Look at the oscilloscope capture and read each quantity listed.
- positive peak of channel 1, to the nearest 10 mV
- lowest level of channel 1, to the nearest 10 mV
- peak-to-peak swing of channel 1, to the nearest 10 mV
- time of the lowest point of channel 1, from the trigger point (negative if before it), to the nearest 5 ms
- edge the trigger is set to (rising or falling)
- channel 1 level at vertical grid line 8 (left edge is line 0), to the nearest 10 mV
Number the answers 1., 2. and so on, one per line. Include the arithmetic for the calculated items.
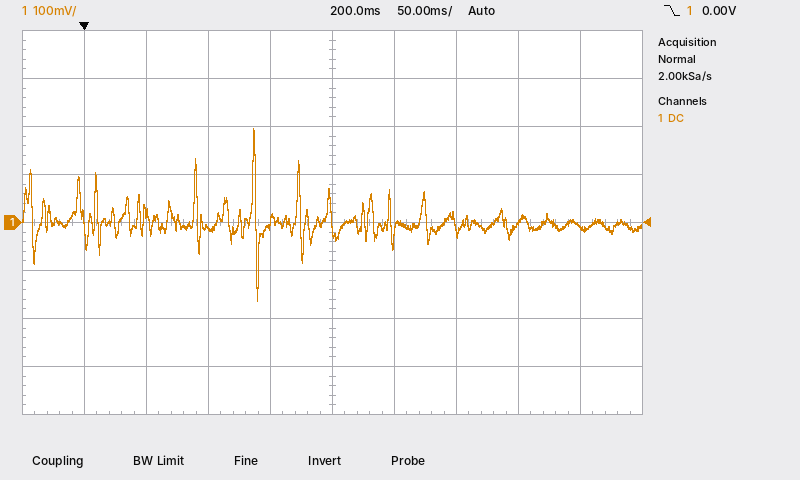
1. 200 mV
2. -160 mV
3. 200 mV − (-160 mV) = 360 mV
4. +140 ms
5. falling
6. 0 mV
